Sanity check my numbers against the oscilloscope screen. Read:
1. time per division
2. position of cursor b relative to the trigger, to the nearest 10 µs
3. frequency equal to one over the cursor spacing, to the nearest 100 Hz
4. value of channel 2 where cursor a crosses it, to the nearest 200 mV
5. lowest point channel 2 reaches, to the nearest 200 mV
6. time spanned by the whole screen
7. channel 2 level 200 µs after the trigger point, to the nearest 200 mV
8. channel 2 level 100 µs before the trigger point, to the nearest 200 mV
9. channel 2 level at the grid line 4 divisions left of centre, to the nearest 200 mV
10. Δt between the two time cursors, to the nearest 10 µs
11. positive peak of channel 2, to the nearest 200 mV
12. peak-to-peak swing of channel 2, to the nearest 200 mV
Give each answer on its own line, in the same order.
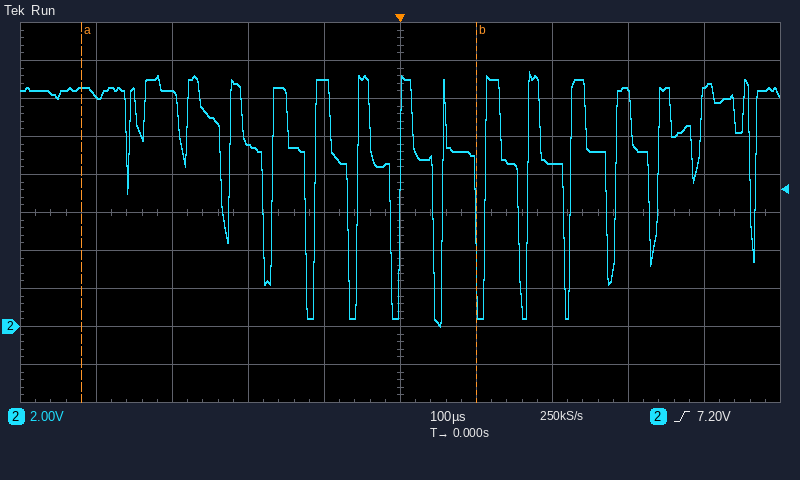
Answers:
100 µs
+100 µs
1.9 kHz
12.6 V
0.0 V
1 ms
8.6 V
13.0 V
12.2 V
520 µs
13.4 V
13.4 V
